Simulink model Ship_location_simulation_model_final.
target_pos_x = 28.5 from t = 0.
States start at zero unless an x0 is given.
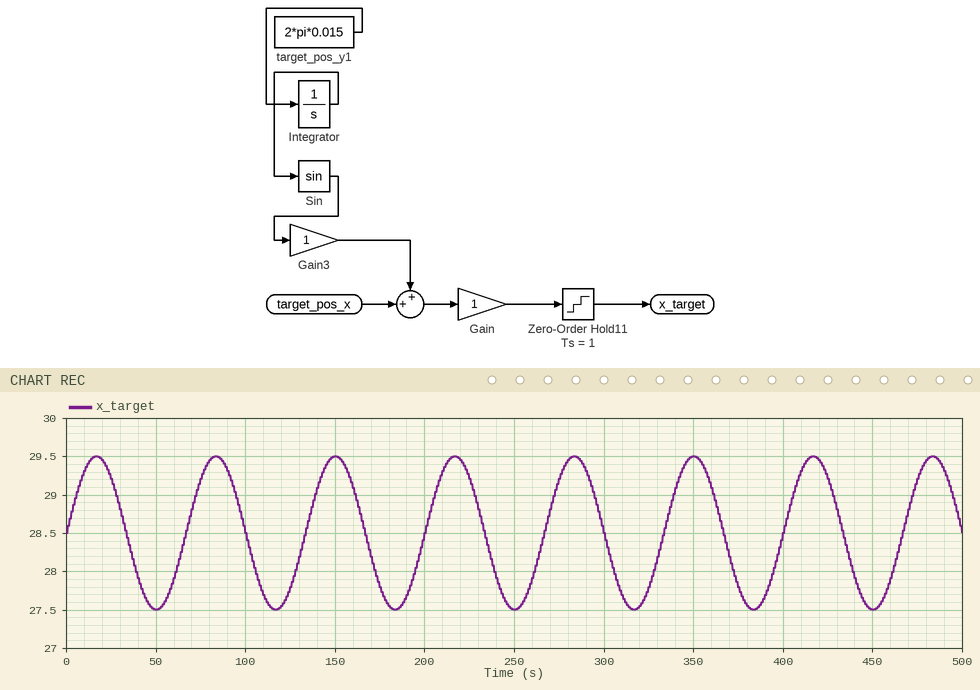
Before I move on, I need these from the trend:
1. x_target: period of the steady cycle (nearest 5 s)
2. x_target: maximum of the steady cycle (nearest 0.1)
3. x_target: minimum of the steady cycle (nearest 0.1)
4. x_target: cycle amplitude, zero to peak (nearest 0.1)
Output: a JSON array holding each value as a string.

["65 s", "29.5", "27.5", "1.0"]
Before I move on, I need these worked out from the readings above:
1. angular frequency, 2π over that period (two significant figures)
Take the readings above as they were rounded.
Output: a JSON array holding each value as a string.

["0.097 rad/s"]
